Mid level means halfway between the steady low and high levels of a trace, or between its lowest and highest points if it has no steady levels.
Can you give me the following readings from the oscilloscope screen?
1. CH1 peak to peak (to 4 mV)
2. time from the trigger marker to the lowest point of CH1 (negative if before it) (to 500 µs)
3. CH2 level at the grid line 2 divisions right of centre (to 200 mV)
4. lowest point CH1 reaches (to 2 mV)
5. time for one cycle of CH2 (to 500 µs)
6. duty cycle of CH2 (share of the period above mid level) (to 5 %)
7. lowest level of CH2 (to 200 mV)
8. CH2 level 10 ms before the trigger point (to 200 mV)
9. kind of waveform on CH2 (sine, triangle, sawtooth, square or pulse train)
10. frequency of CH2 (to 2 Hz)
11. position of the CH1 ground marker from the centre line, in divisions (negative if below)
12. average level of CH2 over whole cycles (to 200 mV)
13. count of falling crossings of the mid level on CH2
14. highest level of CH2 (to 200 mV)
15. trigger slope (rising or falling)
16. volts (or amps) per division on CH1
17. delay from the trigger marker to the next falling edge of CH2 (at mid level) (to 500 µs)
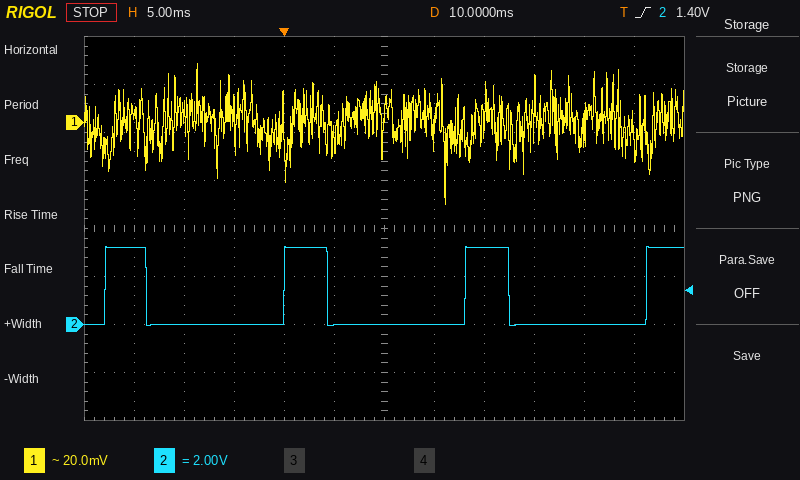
60 mV
+16.0 ms
3.2 V
-34 mV
18.0 ms
25 %
0.0 V
0.0 V
pulse train
56 Hz
+2.2 div
800 mV
3
3.2 V
rising
20 mV
4.5 ms
